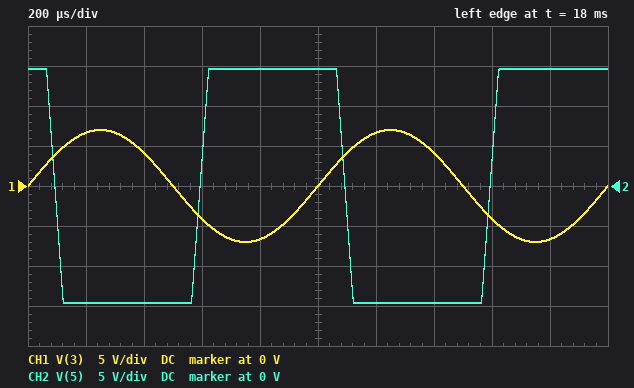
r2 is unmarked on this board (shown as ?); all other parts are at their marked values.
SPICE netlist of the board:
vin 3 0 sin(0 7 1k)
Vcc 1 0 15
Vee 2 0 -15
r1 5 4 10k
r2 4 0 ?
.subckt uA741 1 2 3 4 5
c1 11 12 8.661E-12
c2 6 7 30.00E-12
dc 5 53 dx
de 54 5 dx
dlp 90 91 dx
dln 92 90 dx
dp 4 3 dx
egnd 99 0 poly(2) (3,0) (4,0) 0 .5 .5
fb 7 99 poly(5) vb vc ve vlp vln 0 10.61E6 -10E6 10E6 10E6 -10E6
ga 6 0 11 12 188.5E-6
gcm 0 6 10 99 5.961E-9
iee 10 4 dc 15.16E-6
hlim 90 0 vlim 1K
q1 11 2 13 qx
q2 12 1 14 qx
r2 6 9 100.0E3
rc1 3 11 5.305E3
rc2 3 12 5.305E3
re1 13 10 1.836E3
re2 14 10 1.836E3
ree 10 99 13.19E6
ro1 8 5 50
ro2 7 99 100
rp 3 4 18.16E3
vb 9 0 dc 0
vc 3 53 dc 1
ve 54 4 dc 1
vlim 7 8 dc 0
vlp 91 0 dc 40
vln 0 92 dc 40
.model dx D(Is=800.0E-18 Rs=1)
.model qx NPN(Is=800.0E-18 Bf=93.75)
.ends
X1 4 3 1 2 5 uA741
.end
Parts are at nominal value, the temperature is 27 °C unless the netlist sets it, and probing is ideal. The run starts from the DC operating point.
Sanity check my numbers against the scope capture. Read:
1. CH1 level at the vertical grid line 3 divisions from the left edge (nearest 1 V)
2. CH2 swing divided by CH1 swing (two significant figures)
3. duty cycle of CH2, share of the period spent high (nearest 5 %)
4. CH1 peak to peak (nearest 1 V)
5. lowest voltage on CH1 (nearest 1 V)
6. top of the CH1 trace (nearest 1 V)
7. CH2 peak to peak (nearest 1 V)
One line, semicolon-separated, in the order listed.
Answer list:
-4 V; 2.1; 50 %; 14 V; -7 V; 7 V; 29 V
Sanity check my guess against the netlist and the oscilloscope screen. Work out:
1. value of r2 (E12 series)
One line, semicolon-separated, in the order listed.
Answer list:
2.2 kΩ
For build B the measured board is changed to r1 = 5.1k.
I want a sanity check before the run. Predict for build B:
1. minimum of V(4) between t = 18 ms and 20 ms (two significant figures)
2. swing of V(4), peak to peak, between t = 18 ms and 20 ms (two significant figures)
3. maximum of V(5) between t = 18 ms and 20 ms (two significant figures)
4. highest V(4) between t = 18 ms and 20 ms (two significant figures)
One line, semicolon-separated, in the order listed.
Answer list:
-4.4 V; 8.8 V; 15 V; 4.4 V
